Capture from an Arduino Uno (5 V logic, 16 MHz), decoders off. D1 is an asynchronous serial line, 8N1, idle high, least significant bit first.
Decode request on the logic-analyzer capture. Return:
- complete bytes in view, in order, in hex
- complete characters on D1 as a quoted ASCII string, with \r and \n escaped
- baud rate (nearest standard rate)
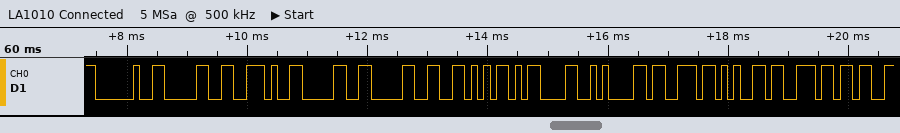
0x20 0x30 0x2E 0x30 0x30 0x56 0x0D 0x0A 0x73 0x65 0x6E
" 0.00V\r\nsen"
9600 baud
